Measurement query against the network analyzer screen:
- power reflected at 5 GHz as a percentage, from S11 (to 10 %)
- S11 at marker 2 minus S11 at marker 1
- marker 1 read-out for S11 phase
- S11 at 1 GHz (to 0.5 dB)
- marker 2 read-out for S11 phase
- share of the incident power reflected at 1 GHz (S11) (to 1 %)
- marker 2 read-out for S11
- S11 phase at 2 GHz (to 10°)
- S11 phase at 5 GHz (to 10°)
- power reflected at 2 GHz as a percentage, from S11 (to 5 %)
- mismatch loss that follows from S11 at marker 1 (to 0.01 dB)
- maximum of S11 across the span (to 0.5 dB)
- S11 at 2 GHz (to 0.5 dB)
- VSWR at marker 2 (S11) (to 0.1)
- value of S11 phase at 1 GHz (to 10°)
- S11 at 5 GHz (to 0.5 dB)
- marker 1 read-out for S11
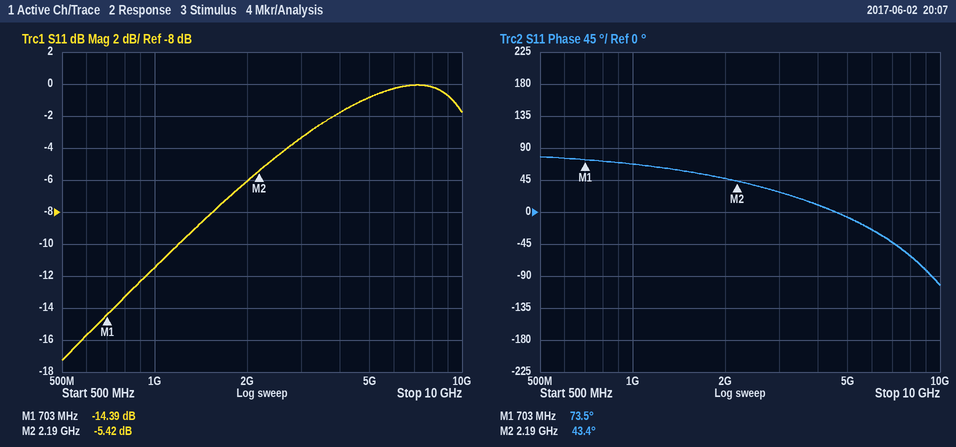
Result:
80 %
8.97 dB
73.5°
-11.5 dB
43.4°
7 %
-5.42 dB
50°
-10°
25 %
0.16 dB
0.0 dB
-6.0 dB
3.3
70°
-1.0 dB
-14.39 dB
